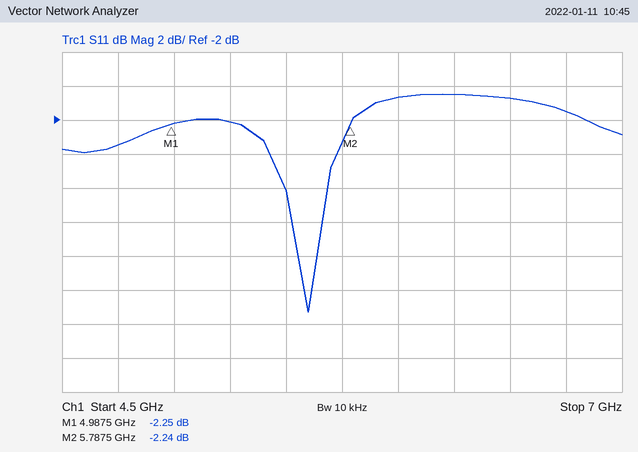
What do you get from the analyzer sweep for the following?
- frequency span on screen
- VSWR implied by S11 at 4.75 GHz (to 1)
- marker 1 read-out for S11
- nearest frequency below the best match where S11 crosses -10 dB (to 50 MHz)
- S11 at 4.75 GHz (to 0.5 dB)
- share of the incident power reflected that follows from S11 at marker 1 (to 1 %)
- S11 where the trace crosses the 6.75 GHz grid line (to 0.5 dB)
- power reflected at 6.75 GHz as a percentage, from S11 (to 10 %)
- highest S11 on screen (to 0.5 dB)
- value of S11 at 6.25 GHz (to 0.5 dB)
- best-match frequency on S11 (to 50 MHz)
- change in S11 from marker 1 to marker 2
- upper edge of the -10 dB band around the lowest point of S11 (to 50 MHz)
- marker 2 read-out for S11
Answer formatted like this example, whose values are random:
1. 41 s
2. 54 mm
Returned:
1. 2.5 GHz
2. 5
3. -2.25 dB
4. 5.55 GHz
5. -3.5 dB
6. 60 %
7. -1.5 dB
8. 70 %
9. -0.5 dB
10. -0.5 dB
11. 5.60 GHz
12. 0.01 dB
13. 5.65 GHz
14. -2.24 dB
